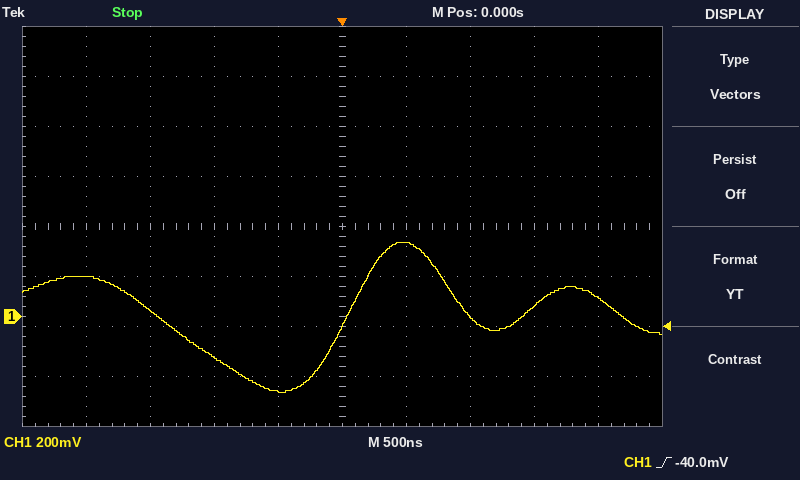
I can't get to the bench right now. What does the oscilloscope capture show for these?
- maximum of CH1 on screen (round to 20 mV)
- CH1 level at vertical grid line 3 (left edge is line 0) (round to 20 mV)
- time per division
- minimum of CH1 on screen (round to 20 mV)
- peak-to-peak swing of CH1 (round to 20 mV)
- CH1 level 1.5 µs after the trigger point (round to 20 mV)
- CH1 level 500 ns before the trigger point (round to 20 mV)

300 mV
-160 mV
500 ns
-300 mV
600 mV
40 mV
-300 mV
